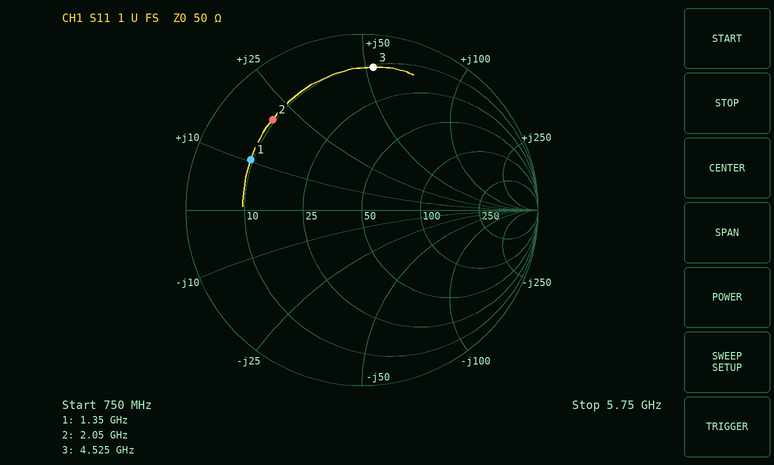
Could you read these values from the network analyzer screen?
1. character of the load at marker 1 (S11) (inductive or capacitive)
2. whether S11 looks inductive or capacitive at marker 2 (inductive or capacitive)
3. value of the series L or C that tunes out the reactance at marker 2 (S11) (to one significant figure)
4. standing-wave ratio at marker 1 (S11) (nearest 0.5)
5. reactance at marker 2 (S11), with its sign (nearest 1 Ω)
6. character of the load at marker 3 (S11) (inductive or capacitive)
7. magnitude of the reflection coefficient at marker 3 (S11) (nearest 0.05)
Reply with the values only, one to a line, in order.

inductive
inductive
4 pF
5.5
+20 Ω
inductive
0.80
